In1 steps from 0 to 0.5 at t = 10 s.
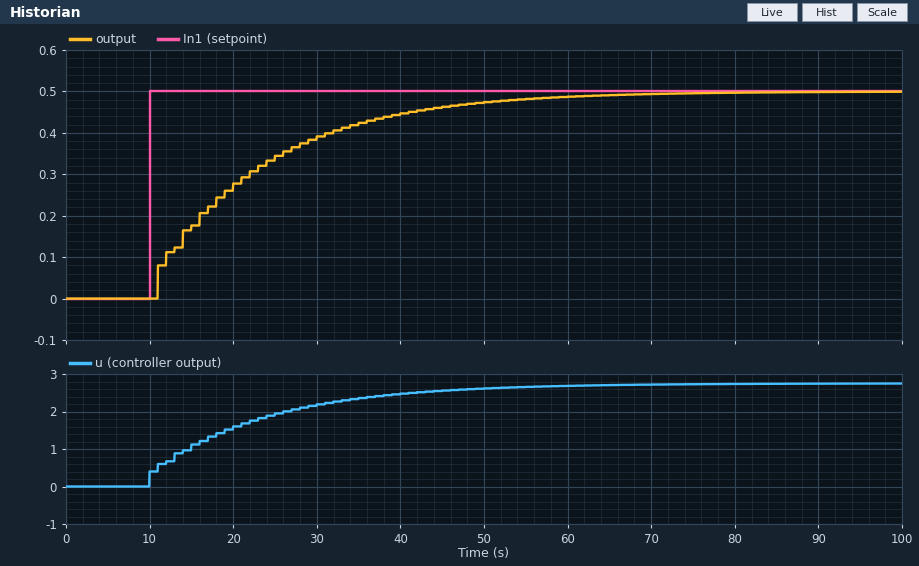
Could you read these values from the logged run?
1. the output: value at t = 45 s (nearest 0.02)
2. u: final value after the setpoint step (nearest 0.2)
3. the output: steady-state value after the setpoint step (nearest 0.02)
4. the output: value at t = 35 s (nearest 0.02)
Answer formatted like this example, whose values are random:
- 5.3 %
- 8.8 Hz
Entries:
- 0.46
- 2.8
- 0.50
- 0.42
